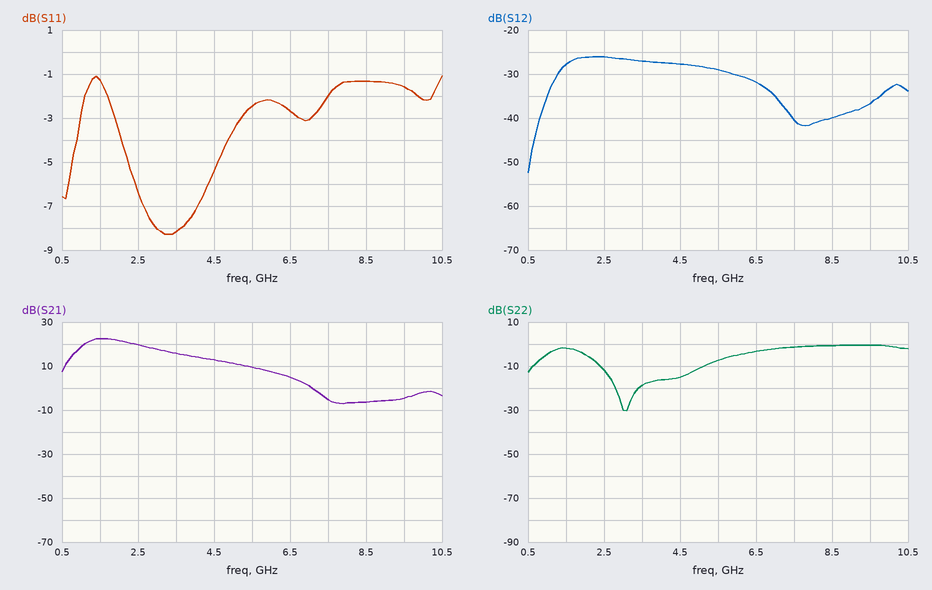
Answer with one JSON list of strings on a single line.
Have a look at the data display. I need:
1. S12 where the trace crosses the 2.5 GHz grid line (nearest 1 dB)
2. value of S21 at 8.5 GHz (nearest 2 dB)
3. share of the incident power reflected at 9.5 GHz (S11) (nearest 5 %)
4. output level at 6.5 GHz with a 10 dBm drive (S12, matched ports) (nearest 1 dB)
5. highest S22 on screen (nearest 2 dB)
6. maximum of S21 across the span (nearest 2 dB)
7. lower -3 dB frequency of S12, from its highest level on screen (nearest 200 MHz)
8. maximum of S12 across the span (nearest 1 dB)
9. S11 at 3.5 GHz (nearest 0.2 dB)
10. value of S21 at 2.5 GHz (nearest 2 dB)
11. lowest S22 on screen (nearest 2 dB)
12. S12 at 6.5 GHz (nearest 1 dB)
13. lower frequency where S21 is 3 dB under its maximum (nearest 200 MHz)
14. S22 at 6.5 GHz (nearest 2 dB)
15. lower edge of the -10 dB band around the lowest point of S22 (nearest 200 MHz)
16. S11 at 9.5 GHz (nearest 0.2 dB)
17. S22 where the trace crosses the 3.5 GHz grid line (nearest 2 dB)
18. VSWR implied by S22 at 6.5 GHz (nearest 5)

["-26 dB", "-6 dB", "70 %", "-22 dBm", "0 dB", "22 dB", "1.4 GHz", "-26 dB", "-8.2 dB", "20 dB", "-30 dB", "-32 dB", "1.0 GHz", "-4 dB", "2.4 GHz", "-1.6 dB", "-18 dB", "5"]
